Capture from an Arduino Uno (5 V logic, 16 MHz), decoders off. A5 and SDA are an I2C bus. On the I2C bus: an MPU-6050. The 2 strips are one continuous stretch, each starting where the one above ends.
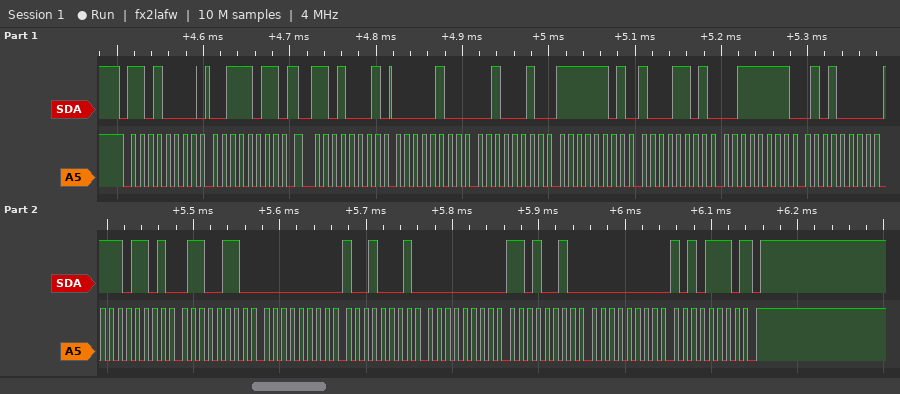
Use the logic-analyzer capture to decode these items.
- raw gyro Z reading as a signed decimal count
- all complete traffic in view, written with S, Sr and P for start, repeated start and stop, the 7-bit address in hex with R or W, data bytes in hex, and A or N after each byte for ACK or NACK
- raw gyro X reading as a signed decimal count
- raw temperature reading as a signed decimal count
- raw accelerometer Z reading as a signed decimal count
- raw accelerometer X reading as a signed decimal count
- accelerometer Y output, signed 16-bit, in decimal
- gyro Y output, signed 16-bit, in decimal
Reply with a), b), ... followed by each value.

a) 174
b) S 68W A 3B A Sr 68R A 04 A 22 A FD A 8D A 3F A 50 A ED A 66 A 00 A 91 A 00 A D2 A 00 A AE N P
c) 145
d) -4762
e) 16208
f) 1058
g) -627
h) 210
